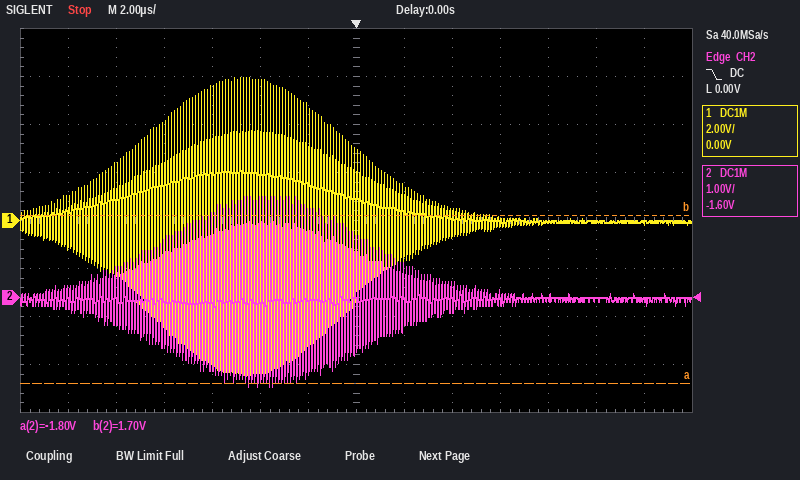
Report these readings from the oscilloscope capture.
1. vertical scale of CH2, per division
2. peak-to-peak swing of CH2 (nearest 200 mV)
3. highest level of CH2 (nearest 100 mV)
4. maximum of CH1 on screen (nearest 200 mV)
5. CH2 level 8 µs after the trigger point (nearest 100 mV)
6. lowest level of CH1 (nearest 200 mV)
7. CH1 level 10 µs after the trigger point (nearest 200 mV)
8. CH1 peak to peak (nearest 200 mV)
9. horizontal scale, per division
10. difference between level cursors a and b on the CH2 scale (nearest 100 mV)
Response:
1 V
4.0 V
2.1 V
6.0 V
0.0 V
-6.4 V
0.0 V
12.4 V
2 µs
3.5 V
